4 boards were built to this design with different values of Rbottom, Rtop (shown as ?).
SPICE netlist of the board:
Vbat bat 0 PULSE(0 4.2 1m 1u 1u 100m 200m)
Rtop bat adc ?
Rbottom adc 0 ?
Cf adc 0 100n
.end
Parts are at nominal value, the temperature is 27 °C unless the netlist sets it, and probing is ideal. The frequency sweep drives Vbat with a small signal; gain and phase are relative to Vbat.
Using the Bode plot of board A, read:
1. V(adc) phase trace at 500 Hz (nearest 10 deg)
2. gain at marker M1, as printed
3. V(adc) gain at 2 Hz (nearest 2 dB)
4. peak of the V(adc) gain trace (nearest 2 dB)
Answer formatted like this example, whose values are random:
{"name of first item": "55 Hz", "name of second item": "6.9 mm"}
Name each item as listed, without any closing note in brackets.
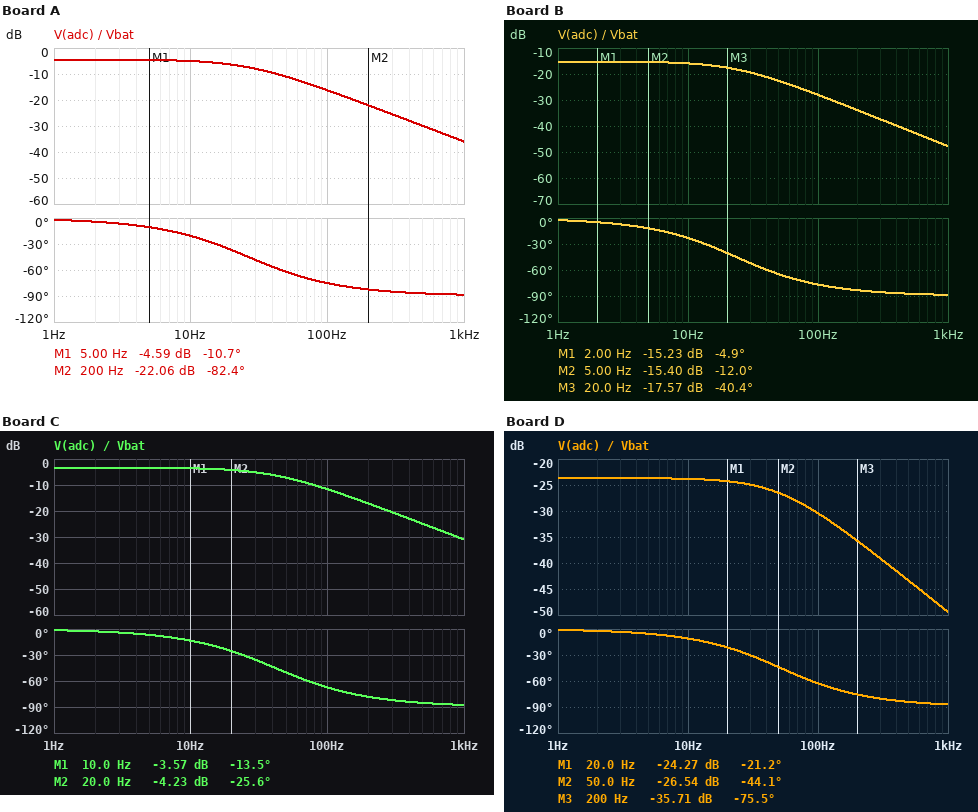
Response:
{"V(adc) phase trace at 500 Hz": "-90 deg", "gain at marker M1, as printed": "-4.59 dB", "V(adc) gain at 2 Hz": "-4 dB", "peak of the V(adc) gain trace": "-4 dB"}
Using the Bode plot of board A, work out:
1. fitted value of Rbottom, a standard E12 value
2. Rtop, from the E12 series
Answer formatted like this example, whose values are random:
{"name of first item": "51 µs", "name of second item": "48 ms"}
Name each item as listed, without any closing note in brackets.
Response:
{"fitted value of Rbottom, a standard E12 value": "150 kΩ", "Rtop, from the E12 series": "100 kΩ"}
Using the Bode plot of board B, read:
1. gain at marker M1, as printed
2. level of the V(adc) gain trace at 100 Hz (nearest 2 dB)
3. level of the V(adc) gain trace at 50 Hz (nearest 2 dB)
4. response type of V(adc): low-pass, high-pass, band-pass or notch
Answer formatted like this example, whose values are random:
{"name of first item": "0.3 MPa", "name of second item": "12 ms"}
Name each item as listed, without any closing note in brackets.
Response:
{"gain at marker M1, as printed": "-15.23 dB", "level of the V(adc) gain trace at 100 Hz": "-28 dB", "level of the V(adc) gain trace at 50 Hz": "-22 dB", "response type of V(adc): low-pass, high-pass, band-pass or notch": "low-pass"}
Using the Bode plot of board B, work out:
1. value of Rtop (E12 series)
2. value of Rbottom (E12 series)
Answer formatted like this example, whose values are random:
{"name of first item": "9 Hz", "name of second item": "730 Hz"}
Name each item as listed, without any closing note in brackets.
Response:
{"value of Rtop": "390 kΩ", "value of Rbottom": "82 kΩ"}
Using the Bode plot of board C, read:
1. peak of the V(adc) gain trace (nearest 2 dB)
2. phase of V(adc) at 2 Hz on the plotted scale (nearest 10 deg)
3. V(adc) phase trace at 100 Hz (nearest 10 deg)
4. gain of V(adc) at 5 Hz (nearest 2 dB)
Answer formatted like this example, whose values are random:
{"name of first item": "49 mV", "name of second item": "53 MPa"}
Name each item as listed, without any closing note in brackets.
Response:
{"peak of the V(adc) gain trace": "-4 dB", "phase of V(adc) at 2 Hz on the plotted scale": "0 deg", "V(adc) phase trace at 100 Hz": "-70 deg", "gain of V(adc) at 5 Hz": "-4 dB"}
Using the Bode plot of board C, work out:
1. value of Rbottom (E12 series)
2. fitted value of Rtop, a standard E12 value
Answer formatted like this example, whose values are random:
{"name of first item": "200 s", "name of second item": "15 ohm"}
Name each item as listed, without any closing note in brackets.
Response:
{"value of Rbottom": "120 kΩ", "fitted value of Rtop, a standard E12 value": "56 kΩ"}
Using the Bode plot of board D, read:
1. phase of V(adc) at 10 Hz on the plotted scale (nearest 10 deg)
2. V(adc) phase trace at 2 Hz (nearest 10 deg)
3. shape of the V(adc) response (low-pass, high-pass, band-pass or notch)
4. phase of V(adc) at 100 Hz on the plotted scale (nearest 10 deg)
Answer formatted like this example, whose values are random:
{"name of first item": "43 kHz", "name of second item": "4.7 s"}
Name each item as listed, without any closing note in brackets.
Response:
{"phase of V(adc) at 10 Hz on the plotted scale": "-10 deg", "V(adc) phase trace at 2 Hz": "0 deg", "shape of the V(adc) response": "low-pass", "phase of V(adc) at 100 Hz on the plotted scale": "-60 deg"}
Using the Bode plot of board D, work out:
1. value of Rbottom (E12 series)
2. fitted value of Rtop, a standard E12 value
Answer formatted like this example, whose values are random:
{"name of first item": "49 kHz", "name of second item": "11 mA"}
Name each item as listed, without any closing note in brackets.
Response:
{"value of Rbottom": "33 kΩ", "fitted value of Rtop, a standard E12 value": "470 kΩ"}
